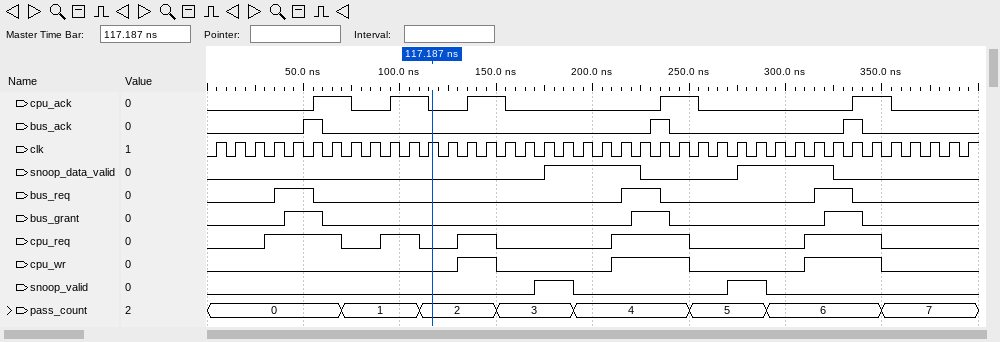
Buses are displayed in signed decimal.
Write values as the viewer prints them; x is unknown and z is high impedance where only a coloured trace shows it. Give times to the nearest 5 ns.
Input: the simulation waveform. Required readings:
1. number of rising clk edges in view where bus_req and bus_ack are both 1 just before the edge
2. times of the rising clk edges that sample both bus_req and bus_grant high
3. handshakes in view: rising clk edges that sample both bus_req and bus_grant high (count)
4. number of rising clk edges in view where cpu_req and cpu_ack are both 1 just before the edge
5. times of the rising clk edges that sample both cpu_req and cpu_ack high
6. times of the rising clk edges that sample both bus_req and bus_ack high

3
45 ns, 55 ns, 225 ns, 235 ns, 325 ns, 335 ns
6
5
65 ns, 105 ns, 145 ns, 245 ns, 345 ns
55 ns, 235 ns, 335 ns
